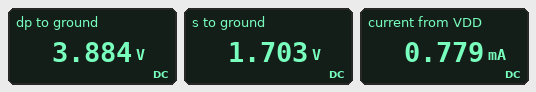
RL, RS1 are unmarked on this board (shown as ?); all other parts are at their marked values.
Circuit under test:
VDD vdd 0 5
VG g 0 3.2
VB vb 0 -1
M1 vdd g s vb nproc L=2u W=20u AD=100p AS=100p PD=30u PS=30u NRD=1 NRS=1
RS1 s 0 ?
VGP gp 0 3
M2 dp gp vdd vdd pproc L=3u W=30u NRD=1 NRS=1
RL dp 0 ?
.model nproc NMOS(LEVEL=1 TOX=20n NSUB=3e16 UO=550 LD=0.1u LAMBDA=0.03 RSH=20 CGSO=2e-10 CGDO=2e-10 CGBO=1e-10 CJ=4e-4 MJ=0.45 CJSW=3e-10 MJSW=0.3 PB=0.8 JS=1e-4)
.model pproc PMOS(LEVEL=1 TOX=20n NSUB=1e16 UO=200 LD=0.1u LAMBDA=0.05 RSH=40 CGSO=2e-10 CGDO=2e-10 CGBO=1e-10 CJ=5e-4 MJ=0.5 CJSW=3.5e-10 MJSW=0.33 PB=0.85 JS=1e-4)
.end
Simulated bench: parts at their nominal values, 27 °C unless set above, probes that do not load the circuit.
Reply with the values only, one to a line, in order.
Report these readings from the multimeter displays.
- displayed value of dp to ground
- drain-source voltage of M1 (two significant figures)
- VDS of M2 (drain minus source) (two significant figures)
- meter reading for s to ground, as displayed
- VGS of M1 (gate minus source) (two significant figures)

3.884 V
3.3 V
-1.1 V
1.703 V
1.5 V
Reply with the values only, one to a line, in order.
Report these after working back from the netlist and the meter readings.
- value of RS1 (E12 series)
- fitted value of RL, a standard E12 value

8.2 kΩ
6.8 kΩ
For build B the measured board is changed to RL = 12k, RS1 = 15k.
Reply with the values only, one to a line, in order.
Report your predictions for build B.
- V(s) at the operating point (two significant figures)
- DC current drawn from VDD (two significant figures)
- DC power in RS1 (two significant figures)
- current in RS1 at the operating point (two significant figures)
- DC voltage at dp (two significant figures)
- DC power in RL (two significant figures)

1.8 V
490 µA
220 µW
120 µA
4.4 V
1.6 mW
